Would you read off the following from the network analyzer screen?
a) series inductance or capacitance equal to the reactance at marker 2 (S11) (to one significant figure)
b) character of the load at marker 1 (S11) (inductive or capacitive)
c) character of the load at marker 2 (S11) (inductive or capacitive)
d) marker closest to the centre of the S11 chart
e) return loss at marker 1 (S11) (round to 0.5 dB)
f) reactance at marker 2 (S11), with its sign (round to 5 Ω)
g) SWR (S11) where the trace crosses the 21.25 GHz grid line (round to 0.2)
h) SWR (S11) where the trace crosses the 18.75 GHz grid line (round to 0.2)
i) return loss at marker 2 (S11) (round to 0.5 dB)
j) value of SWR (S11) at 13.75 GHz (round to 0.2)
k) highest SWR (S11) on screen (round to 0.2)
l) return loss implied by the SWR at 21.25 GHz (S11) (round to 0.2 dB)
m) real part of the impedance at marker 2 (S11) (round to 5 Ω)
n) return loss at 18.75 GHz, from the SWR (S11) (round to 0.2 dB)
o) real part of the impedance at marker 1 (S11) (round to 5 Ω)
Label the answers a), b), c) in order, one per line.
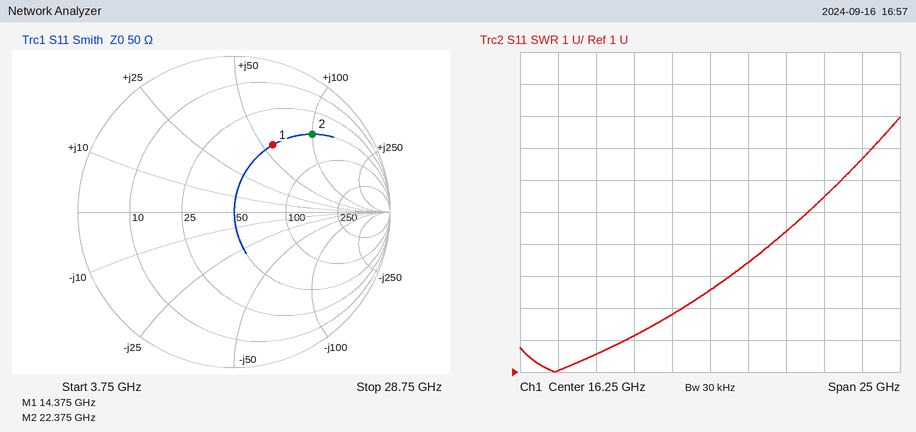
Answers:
a) 700 pH
b) inductive
c) inductive
d) marker 1
e) 6.0 dB
f) +100 Ω
g) 5.4
h) 4.4
i) 3.0 dB
j) 2.8
k) 9.0
l) 3.2 dB
m) 50 Ω
n) 4.0 dB
o) 50 Ω
